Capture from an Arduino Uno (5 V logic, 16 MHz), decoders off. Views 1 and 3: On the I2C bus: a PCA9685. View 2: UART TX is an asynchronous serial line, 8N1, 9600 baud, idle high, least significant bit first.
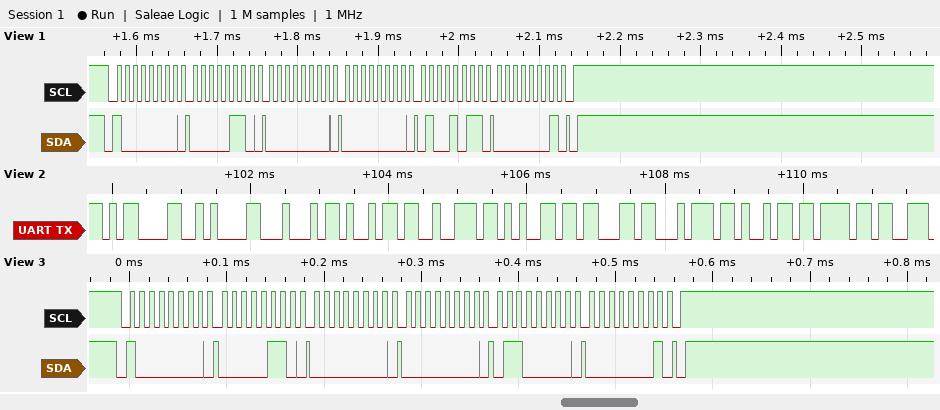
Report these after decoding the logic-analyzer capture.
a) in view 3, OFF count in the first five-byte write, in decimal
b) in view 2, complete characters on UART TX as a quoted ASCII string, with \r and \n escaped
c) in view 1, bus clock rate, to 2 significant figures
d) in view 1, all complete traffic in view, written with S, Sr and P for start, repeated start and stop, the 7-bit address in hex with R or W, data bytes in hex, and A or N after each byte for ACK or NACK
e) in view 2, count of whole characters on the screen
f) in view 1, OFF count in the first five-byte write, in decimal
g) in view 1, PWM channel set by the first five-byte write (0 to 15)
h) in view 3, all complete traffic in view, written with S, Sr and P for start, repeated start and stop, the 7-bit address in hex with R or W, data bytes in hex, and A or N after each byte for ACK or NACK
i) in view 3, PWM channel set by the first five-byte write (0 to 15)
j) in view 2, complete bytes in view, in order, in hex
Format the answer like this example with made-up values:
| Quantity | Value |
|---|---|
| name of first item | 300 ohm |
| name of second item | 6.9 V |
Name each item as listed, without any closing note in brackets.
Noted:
| Quantity | Value |
|---|---|
| in view 3, OFF count in the first five-byte write, in decimal | 352 |
| in view 2, complete characters on UART TX as a quoted ASCII string, with \r and \n escaped | "\r\nDirectio" |
| in view 1, bus clock rate, to 2 significant figures | 100 kHz |
| in view 1, all complete traffic in view, written with S, Sr and P for start, repeated start and stop, the 7-bit address in hex with R or W, data bytes in hex, and A or N after each byte for ACK or NACK | S 40W A 06 A 00 A 00 A 4B A 01 A P |
| in view 2, count of whole characters on the screen | 10 |
| in view 1, OFF count in the first five-byte write, in decimal | 331 |
| in view 1, PWM channel set by the first five-byte write | 0 |
| in view 3, all complete traffic in view, written with S, Sr and P for start, repeated start and stop, the 7-bit address in hex with R or W, data bytes in hex, and A or N after each byte for ACK or NACK | S 40W A 06 A 00 A 00 A 60 A 01 A P |
| in view 3, PWM channel set by the first five-byte write | 0 |
| in view 2, complete bytes in view, in order, in hex | 0D 0A 44 69 72 65 63 74 69 6F |
